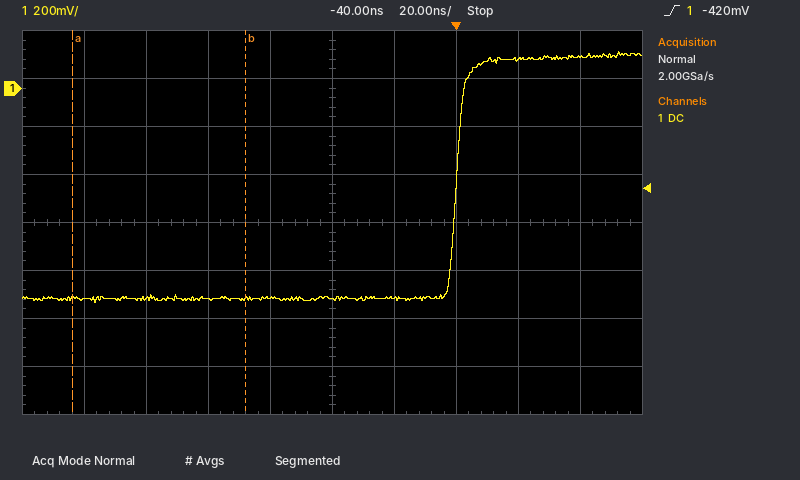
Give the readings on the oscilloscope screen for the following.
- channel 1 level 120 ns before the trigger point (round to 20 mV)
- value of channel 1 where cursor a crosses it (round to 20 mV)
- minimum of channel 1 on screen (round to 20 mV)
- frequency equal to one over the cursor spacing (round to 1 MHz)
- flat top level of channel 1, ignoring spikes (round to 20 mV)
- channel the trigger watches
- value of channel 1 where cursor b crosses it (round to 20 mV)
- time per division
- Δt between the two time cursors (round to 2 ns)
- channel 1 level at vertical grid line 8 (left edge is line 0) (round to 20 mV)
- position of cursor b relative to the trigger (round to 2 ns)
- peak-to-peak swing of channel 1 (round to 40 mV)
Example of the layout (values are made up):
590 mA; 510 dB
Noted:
-880 mV; -880 mV; -900 mV; 18 MHz; 120 mV; channel 1; -880 mV; 20 ns; 56 ns; 120 mV; -68 ns; 1.04 V
